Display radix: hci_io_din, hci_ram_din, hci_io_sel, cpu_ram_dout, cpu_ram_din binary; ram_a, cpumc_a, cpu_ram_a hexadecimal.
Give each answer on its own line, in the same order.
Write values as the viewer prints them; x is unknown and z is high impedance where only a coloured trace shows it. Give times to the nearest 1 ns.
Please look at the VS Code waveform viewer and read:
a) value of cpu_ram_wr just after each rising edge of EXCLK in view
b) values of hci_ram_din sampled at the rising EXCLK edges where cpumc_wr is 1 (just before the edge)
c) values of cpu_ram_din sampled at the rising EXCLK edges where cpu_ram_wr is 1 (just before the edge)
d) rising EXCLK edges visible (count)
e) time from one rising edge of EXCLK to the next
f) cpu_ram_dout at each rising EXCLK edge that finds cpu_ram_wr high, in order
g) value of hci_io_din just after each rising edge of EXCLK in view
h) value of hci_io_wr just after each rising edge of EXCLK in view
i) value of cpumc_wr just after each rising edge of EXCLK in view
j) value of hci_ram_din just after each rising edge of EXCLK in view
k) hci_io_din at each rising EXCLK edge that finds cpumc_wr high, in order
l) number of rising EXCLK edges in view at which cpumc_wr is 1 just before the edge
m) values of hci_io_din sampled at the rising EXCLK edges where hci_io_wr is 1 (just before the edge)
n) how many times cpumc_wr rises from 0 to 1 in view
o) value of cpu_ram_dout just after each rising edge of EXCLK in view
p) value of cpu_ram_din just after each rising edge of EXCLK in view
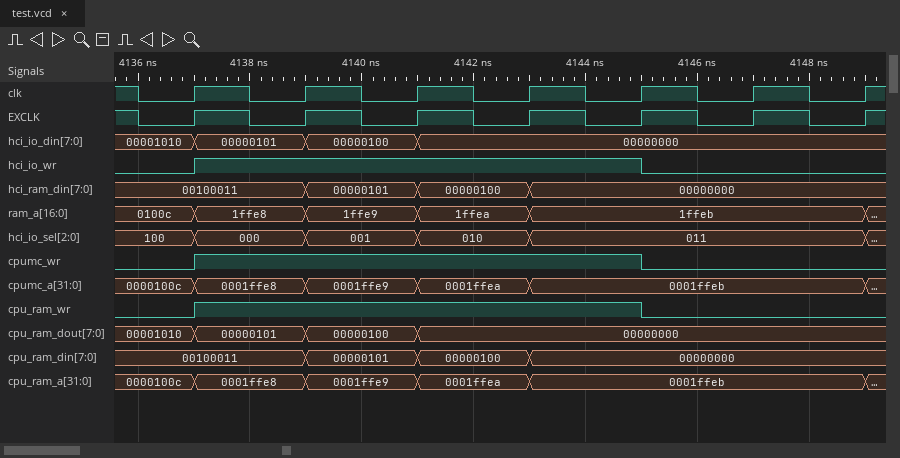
1 1 1 1 0 0 0
00100011, 00000101, 00000100, 00000000
00100011, 00000101, 00000100, 00000000
7
2 ns
00000101, 00000100, 00000000, 00000000
00000101, 00000100, 00000000, 00000000, 00000000, 00000000, 00000000
1 1 1 1 0 0 0
1 1 1 1 0 0 0
00100011, 00000101, 00000100, 00000000, 00000000, 00000000, 00000000
00000101, 00000100, 00000000, 00000000
4
00000101, 00000100, 00000000, 00000000
1
00000101, 00000100, 00000000, 00000000, 00000000, 00000000, 00000000
00100011, 00000101, 00000100, 00000000, 00000000, 00000000, 00000000
